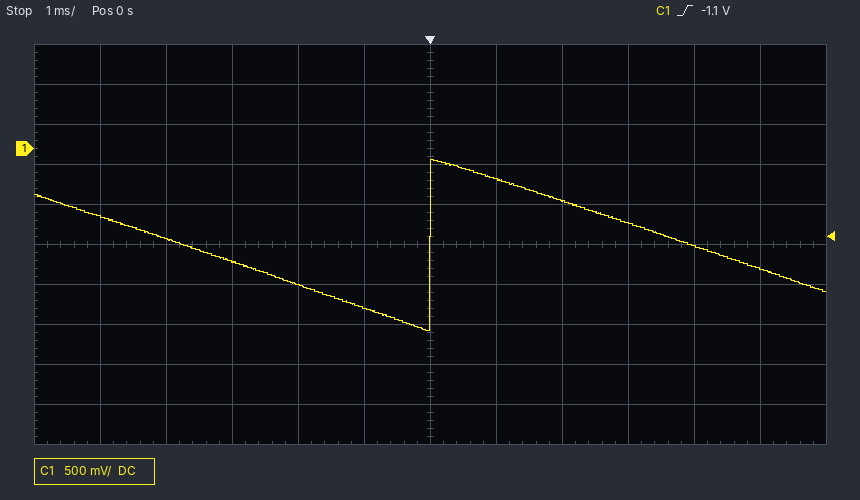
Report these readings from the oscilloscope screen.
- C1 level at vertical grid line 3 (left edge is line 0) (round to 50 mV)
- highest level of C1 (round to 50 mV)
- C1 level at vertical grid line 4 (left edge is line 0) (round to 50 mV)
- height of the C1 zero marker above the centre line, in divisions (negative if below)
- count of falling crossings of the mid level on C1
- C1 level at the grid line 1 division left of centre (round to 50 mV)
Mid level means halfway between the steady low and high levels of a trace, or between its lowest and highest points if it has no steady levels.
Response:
-1.40 V
-150 mV
-1.70 V
+2.4 div
2
-2.00 V
